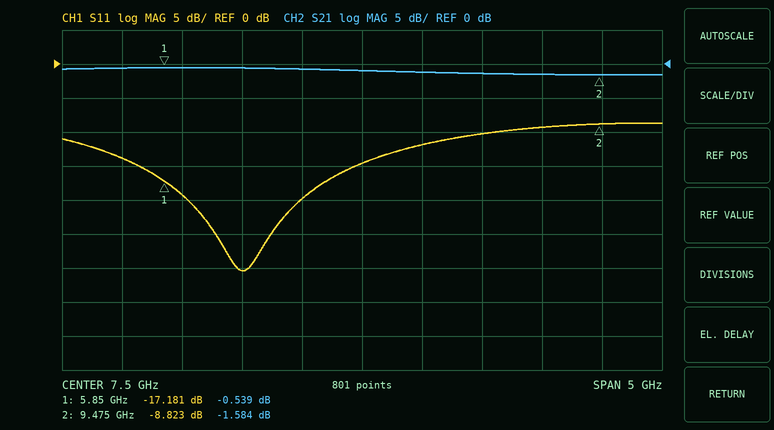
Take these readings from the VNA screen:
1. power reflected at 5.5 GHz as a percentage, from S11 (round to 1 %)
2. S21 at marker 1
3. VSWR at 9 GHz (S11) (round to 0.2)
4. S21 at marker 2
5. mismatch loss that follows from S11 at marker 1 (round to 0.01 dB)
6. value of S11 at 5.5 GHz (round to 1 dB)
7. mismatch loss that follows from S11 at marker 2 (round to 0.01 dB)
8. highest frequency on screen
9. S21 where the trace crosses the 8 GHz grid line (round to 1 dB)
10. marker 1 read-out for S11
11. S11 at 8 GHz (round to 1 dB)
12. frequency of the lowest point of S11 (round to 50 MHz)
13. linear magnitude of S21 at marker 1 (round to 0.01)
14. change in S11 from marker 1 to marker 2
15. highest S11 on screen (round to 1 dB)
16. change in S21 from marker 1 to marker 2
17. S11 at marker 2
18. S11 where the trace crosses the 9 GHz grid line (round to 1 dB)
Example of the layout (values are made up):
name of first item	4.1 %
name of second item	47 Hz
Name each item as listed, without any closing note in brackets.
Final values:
power reflected at 5.5 GHz as a percentage, from S11	4 %
S21 at marker 1	-0.539 dB
VSWR at 9 GHz (S11)	2.0
S21 at marker 2	-1.584 dB
mismatch loss that follows from S11 at marker 1	0.08 dB
value of S11 at 5.5 GHz	-14 dB
mismatch loss that follows from S11 at marker 2	0.61 dB
highest frequency on screen	10 GHz
S21 where the trace crosses the 8 GHz grid line	-1 dB
marker 1 read-out for S11	-17.181 dB
S11 at 8 GHz	-12 dB
frequency of the lowest point of S11	6.50 GHz
linear magnitude of S21 at marker 1	0.94
change in S11 from marker 1 to marker 2	8.358 dB
highest S11 on screen	-9 dB
change in S21 from marker 1 to marker 2	-1.045 dB
S11 at marker 2	-8.823 dB
S11 where the trace crosses the 9 GHz grid line	-9 dB
